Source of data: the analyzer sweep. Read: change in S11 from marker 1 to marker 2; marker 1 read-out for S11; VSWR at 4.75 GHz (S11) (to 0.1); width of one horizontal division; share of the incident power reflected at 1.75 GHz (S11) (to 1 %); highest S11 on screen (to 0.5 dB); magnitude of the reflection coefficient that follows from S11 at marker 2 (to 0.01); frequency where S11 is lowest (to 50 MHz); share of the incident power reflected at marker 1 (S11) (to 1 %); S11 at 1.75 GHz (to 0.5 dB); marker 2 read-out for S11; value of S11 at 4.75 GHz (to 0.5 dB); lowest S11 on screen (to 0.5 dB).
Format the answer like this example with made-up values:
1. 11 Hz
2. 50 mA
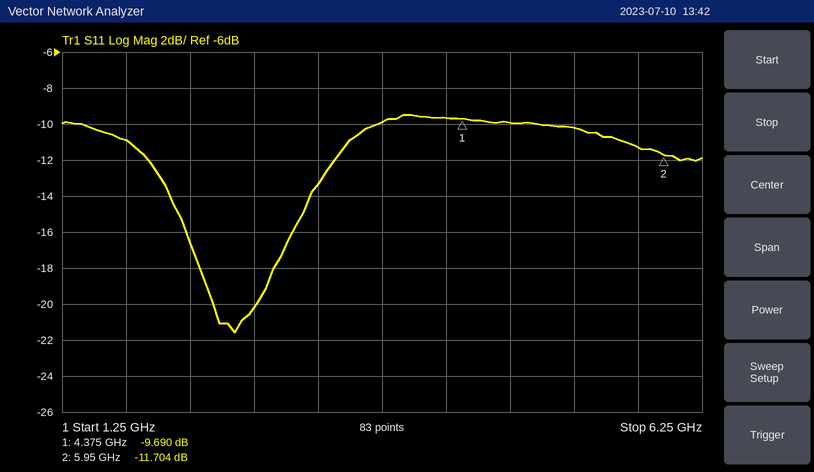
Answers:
1. -2.014 dB
2. -9.690 dB
3. 1.9
4. 500 MHz
5. 8 %
6. -9.5 dB
7. 0.26
8. 2.60 GHz
9. 11 %
10. -11.0 dB
11. -11.704 dB
12. -10.0 dB
13. -21.5 dB
